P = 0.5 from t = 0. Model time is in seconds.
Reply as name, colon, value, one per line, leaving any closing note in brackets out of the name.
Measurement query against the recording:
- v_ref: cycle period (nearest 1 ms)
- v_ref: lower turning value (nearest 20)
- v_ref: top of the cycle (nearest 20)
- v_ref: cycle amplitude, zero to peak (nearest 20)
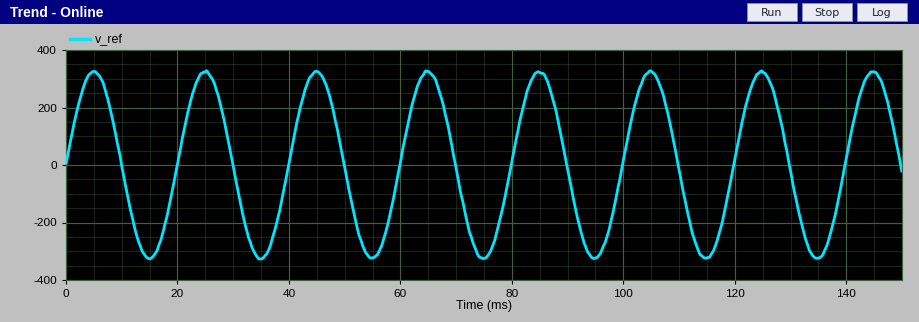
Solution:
v_ref: cycle period: 20 ms
v_ref: lower turning value: -320
v_ref: top of the cycle: 320
v_ref: cycle amplitude, zero to peak: 320
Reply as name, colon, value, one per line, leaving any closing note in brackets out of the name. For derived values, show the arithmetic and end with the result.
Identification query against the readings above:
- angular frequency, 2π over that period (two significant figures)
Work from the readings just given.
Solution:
angular frequency, 2π over that period: 2π / 20 = 0.31 rad/ms
